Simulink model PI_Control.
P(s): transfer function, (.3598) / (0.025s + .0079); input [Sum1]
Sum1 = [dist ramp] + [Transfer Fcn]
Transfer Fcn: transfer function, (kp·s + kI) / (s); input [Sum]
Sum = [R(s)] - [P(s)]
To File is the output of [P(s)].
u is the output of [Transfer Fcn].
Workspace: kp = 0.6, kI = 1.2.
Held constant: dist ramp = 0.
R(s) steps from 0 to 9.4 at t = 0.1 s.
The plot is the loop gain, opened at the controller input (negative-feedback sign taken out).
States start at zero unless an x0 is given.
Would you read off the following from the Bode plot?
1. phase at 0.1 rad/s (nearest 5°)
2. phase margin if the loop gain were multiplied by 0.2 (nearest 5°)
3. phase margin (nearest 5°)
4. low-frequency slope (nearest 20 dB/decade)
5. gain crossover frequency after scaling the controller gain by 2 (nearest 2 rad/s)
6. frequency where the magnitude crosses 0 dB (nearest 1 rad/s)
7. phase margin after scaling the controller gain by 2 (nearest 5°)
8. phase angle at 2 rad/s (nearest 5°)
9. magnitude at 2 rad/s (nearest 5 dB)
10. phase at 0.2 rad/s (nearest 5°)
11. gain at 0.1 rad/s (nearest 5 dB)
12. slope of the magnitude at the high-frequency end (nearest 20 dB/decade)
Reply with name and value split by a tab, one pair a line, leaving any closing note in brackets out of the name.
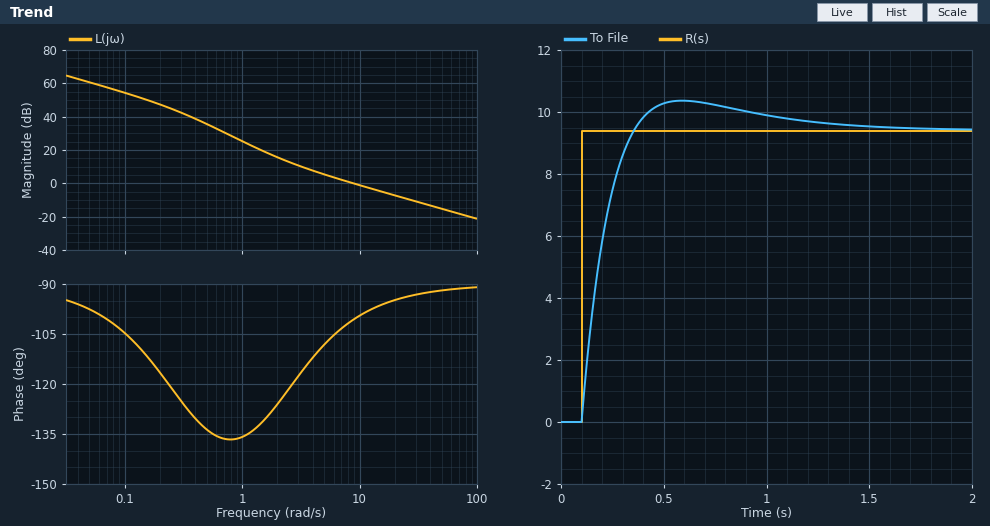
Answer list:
phase at 0.1 rad/s	-105°
phase margin if the loop gain were multiplied by 0.2	55°
phase margin	80°
low-frequency slope	-20 dB/decade
gain crossover frequency after scaling the controller gain by 2	18 rad/s
frequency where the magnitude crosses 0 dB	9 rad/s
phase margin after scaling the controller gain by 2	85°
phase angle at 2 rad/s	-125°
magnitude at 2 rad/s	15 dB
phase at 0.2 rad/s	-115°
gain at 0.1 rad/s	55 dB
slope of the magnitude at the high-frequency end	-20 dB/decade
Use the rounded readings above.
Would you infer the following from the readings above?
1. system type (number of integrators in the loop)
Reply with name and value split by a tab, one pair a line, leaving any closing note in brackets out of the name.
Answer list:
system type	1
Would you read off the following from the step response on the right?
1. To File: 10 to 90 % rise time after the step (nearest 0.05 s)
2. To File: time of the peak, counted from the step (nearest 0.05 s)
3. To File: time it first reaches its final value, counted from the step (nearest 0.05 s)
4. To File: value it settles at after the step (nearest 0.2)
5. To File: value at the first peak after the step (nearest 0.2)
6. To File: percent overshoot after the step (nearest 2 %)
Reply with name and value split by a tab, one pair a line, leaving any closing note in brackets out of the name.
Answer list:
To File: 10 to 90 % rise time after the step	0.20 s
To File: time of the peak, counted from the step	0.50 s
To File: time it first reaches its final value, counted from the step	0.25 s
To File: value it settles at after the step	9.4
To File: value at the first peak after the step	10.4
To File: percent overshoot after the step	10 %
